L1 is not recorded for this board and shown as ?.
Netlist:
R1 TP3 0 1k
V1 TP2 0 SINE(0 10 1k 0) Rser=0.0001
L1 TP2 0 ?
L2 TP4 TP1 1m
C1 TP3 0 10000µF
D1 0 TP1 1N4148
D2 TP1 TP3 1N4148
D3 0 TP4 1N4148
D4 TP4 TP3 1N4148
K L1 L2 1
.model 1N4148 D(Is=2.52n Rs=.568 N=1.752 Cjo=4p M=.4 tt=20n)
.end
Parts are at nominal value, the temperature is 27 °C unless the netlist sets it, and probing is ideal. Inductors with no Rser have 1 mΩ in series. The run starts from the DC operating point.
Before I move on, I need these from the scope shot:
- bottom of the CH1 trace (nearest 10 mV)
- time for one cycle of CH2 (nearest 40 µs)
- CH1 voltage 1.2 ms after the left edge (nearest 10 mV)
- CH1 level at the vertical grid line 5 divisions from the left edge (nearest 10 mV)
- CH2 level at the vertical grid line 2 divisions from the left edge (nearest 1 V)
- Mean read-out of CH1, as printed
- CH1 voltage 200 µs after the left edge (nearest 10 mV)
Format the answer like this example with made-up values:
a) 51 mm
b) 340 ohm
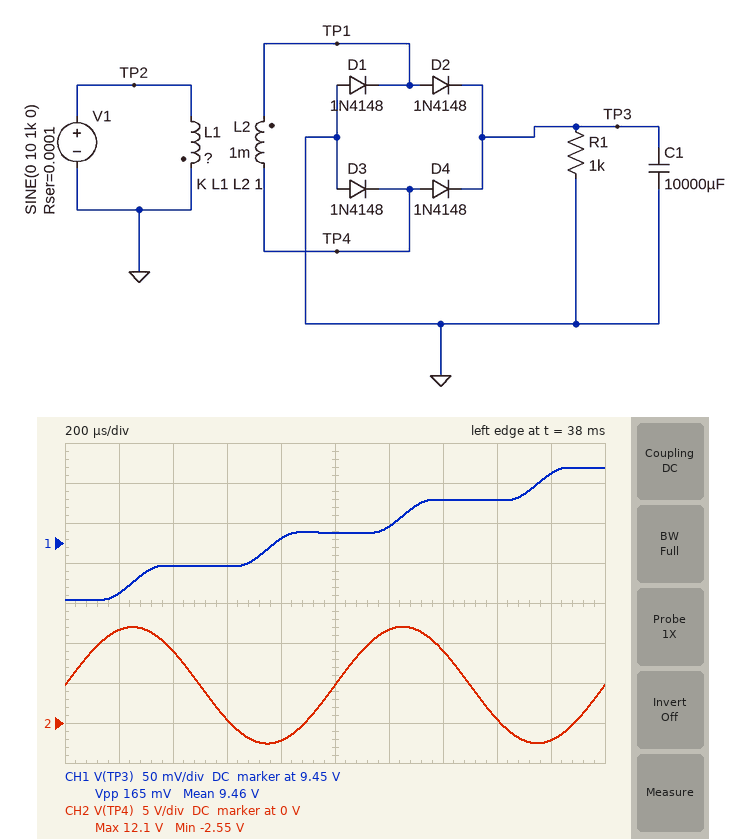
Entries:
a) 9.38 V
b) 1.00 ms
c) 9.47 V
d) 9.46 V
e) 9 V
f) 9.46 V
g) 9.39 V
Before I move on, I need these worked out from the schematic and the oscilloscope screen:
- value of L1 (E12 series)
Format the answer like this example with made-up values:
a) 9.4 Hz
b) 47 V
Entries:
a) 470 µH
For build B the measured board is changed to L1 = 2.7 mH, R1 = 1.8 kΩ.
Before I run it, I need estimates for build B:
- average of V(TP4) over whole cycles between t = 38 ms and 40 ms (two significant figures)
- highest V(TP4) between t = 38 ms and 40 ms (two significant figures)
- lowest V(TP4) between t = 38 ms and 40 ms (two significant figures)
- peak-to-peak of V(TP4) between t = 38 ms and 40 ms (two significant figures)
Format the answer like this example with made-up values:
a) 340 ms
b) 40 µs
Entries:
a) 1.5 V
b) 4.6 V
c) -1.5 V
d) 6.1 V
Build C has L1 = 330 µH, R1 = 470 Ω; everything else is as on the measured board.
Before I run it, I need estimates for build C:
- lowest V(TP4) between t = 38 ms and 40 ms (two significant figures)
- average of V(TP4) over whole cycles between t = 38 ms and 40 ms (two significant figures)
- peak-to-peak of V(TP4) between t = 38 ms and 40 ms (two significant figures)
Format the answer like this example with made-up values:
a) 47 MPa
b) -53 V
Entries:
a) -2.9 V
b) 5.8 V
c) 17 V
